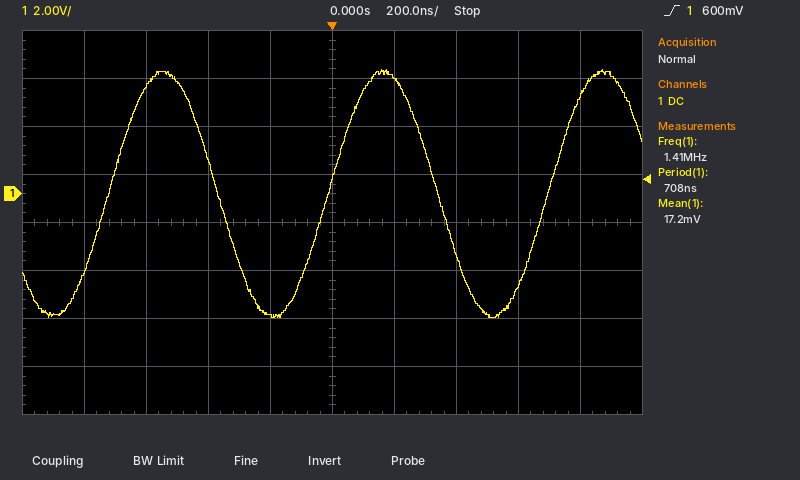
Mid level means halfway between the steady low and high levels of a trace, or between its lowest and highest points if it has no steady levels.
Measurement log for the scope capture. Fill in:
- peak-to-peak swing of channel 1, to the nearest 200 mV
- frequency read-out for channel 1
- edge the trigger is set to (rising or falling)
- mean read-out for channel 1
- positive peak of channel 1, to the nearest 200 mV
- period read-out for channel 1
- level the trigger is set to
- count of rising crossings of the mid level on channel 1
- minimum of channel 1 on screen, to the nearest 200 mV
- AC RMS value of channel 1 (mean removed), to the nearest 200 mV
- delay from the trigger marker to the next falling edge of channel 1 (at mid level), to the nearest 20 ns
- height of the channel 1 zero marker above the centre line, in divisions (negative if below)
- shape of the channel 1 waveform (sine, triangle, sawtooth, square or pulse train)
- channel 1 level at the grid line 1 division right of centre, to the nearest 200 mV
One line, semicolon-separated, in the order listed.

10.4 V; 1.41 MHz; rising; 17.2 mV; 5.2 V; 708 ns; 600 mV; 3; -5.2 V; 3.6 V; 340 ns; +0.6 div; sine; 4.8 V
